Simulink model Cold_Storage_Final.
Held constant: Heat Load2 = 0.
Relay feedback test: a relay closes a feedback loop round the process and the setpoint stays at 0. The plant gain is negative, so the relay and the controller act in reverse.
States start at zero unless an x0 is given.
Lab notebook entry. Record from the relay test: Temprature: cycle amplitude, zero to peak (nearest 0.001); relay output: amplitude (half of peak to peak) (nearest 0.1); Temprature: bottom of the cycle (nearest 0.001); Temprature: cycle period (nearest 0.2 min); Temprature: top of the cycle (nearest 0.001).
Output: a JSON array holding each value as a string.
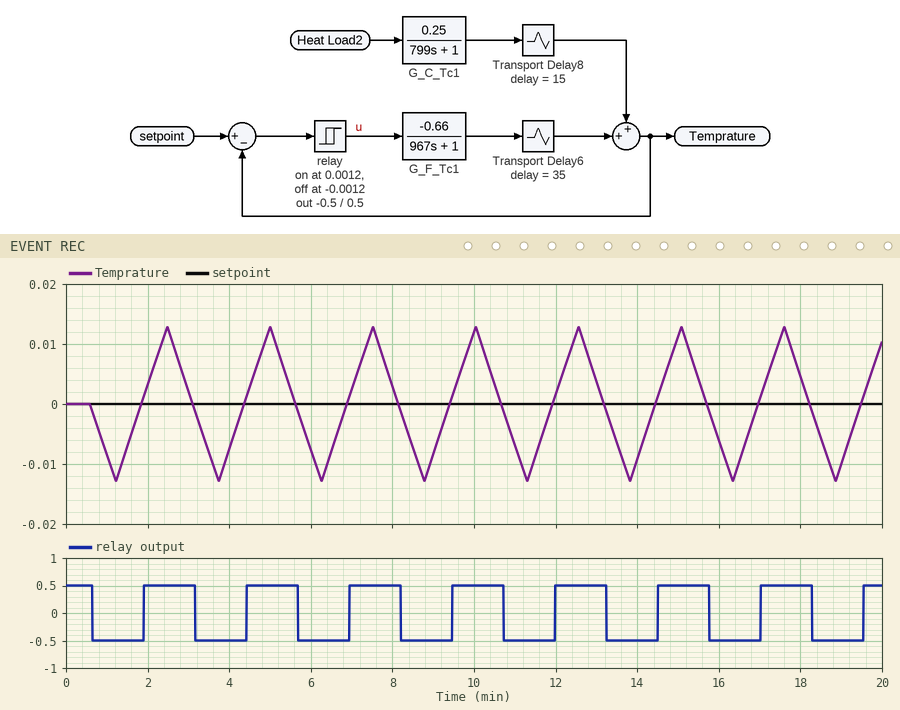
["0.013", "0.5", "-0.013", "2.6 min", "0.013"]
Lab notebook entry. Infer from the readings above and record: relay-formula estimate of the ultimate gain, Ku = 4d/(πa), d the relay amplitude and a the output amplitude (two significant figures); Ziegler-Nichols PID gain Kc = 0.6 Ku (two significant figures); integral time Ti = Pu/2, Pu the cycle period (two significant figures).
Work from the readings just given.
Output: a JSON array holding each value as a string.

["49", "29", "1.3 min"]
